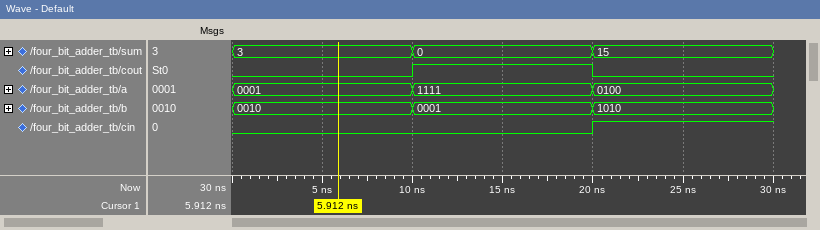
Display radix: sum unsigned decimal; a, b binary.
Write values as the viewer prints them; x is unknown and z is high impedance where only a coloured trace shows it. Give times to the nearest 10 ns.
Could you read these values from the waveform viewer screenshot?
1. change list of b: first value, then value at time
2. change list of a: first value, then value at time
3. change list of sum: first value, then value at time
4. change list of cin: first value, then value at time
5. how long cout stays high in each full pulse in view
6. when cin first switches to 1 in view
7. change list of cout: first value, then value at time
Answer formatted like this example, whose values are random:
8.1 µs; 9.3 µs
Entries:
0010, 0001 at 10 ns, 1010 at 20 ns; 0001, 1111 at 10 ns, 0100 at 20 ns; 3, 0 at 10 ns, 15 at 20 ns; 0, 1 at 20 ns; 10 ns; 20 ns; 0, 1 at 10 ns, 0 at 20 ns
